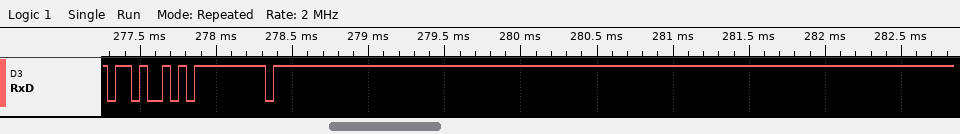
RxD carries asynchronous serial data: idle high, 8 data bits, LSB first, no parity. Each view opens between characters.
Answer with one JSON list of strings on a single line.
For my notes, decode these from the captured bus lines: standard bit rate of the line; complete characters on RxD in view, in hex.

["19200 baud", "4B, FF, FF"]
